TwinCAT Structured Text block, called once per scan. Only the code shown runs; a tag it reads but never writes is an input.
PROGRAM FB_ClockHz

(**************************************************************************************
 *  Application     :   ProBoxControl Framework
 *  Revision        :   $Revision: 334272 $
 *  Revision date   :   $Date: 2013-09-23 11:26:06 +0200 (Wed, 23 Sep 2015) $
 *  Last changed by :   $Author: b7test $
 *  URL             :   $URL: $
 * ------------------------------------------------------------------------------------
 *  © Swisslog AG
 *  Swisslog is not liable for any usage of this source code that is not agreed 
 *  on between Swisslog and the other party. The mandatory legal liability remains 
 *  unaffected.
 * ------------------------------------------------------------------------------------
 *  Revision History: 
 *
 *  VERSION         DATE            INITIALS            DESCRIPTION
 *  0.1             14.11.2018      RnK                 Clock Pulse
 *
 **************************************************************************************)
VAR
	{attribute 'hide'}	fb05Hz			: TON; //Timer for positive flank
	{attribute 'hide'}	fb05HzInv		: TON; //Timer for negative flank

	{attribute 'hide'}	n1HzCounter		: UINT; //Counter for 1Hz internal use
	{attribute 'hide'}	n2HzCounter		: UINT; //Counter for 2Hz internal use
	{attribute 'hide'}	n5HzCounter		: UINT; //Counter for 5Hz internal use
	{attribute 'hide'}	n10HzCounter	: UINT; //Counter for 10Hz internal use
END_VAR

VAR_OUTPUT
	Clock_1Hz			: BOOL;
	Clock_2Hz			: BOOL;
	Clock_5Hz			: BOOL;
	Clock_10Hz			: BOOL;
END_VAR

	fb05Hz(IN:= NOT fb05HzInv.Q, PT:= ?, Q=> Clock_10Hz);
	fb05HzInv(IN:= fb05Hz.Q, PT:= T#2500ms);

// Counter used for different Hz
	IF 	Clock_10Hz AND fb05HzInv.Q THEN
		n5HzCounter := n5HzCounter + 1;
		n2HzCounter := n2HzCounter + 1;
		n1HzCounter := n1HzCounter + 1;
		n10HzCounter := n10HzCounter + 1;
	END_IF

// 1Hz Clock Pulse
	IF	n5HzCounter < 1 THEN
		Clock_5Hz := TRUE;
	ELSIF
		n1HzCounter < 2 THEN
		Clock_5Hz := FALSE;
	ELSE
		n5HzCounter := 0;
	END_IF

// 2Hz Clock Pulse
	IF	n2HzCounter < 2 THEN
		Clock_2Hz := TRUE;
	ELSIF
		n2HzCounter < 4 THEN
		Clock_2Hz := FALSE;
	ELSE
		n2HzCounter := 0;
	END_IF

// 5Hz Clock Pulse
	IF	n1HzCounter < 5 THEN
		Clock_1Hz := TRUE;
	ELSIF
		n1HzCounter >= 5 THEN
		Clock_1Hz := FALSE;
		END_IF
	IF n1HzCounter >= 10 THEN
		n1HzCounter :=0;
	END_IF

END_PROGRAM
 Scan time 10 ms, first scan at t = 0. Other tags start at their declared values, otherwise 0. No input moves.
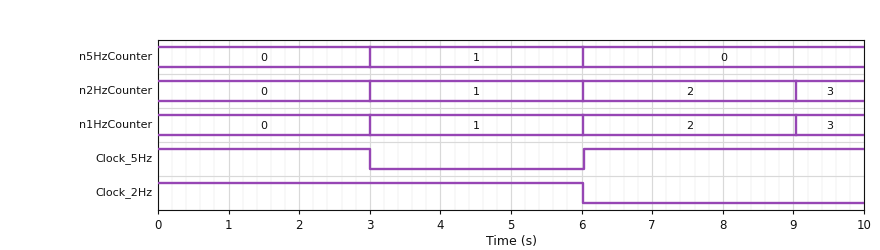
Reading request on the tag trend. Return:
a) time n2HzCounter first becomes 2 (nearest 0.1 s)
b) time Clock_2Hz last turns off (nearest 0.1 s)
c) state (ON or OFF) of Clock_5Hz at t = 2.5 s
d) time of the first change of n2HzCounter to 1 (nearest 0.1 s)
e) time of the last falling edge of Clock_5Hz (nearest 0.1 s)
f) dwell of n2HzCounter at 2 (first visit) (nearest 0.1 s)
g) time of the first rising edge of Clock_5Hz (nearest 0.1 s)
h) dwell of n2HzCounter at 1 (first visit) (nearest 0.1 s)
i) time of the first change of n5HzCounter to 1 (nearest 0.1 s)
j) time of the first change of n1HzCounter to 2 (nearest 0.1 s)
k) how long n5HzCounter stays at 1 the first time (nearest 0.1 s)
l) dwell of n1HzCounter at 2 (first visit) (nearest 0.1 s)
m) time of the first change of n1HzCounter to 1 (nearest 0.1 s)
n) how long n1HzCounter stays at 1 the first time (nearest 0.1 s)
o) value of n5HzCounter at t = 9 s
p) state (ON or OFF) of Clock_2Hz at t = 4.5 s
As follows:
6.0 s
6.0 s
ON
3.0 s
3.0 s
3.0 s
6.0 s
3.0 s
3.0 s
6.0 s
3.0 s
3.0 s
3.0 s
3.0 s
0
ON
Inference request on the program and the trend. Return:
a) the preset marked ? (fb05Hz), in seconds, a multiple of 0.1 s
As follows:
0.5 s
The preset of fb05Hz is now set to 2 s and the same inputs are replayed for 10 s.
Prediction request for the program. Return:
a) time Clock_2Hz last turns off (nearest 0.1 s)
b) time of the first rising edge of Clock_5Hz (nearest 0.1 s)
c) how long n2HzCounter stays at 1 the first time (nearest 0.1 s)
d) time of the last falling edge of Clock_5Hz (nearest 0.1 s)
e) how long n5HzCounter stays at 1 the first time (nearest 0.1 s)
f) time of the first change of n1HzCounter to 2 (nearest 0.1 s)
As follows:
9.0 s
9.0 s
4.5 s
4.5 s
4.5 s
9.0 s
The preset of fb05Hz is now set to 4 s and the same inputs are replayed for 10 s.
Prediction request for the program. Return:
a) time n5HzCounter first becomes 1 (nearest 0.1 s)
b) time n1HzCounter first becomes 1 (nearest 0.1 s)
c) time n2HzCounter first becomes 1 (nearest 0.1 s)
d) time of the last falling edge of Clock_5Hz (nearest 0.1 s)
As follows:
6.5 s
6.5 s
6.5 s
6.5 s
